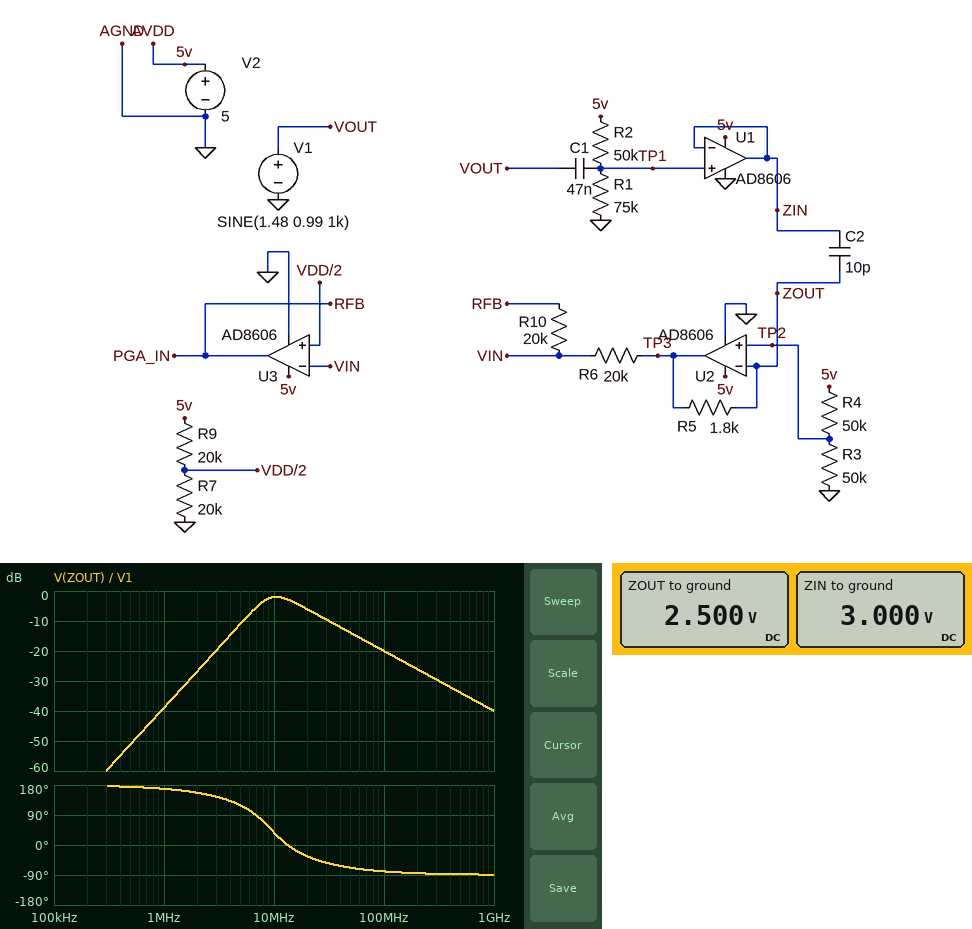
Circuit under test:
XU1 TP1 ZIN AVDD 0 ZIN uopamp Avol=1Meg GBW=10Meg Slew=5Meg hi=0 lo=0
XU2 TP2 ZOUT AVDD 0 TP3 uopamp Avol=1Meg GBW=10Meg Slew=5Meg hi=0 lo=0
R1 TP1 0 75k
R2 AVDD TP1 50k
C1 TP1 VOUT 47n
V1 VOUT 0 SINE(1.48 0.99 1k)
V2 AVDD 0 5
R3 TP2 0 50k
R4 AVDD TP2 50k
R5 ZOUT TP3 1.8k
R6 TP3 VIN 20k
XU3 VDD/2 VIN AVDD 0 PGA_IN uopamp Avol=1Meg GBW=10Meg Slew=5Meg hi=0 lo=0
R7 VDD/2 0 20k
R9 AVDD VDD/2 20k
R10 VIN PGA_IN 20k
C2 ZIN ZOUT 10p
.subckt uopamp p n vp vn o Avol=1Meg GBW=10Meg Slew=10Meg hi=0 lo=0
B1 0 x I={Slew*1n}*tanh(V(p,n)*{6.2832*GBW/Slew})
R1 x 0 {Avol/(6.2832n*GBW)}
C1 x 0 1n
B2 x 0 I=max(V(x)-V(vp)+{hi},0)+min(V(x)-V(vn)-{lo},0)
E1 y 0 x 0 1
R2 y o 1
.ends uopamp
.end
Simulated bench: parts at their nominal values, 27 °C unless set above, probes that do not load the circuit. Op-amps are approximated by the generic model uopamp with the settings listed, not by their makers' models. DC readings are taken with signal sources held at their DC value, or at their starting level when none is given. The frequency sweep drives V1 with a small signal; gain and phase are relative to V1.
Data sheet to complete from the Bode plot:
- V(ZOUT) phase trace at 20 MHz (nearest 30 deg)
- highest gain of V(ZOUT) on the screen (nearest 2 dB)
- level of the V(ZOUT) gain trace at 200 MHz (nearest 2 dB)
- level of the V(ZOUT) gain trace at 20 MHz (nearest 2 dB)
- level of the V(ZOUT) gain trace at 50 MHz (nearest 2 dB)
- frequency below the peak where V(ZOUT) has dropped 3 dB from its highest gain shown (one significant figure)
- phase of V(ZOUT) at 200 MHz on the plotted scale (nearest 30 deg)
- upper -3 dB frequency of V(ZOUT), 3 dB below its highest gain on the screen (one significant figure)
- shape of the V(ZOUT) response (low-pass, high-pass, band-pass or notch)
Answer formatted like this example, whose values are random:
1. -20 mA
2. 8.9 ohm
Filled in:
1. -30 deg
2. -2 dB
3. -26 dB
4. -6 dB
5. -14 dB
6. 7 MHz
7. -90 deg
8. 20 MHz
9. band-pass
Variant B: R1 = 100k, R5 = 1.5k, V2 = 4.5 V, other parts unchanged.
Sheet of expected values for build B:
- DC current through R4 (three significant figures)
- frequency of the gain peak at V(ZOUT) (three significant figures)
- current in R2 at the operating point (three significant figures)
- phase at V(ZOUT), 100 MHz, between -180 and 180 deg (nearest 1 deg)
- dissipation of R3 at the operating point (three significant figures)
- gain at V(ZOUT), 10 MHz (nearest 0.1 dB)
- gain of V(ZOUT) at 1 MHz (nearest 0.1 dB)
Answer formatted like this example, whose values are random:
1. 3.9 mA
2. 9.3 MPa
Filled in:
1. 45.0 µA
2. 11.6 MHz
3. 30.0 µA
4. -78 deg
5. 101 µW
6. -3.5 dB
7. -40.5 dB
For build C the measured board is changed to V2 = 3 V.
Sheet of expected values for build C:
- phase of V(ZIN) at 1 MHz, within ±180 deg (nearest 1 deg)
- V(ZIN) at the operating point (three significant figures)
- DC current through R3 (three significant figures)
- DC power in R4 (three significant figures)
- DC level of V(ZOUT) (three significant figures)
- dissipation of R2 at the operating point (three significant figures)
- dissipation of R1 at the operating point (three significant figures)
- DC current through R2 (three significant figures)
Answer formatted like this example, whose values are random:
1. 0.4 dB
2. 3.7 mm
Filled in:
1. -6 deg
2. 1.80 V
3. 30.0 µA
4. 45.0 µW
5. 1.50 V
6. 28.8 µW
7. 43.2 µW
8. 24.0 µA
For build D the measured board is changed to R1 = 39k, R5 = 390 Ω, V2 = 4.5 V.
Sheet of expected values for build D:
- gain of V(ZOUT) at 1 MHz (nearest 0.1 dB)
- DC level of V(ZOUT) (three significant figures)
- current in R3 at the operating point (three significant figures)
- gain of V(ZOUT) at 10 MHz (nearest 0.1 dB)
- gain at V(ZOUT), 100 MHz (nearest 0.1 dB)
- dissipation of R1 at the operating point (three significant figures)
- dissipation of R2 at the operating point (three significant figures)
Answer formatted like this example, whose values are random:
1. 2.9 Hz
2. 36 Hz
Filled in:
1. -52.3 dB
2. 2.25 V
3. 45.0 µA
4. -17.2 dB
5. -20.4 dB
6. 99.7 µW
7. 128 µW
